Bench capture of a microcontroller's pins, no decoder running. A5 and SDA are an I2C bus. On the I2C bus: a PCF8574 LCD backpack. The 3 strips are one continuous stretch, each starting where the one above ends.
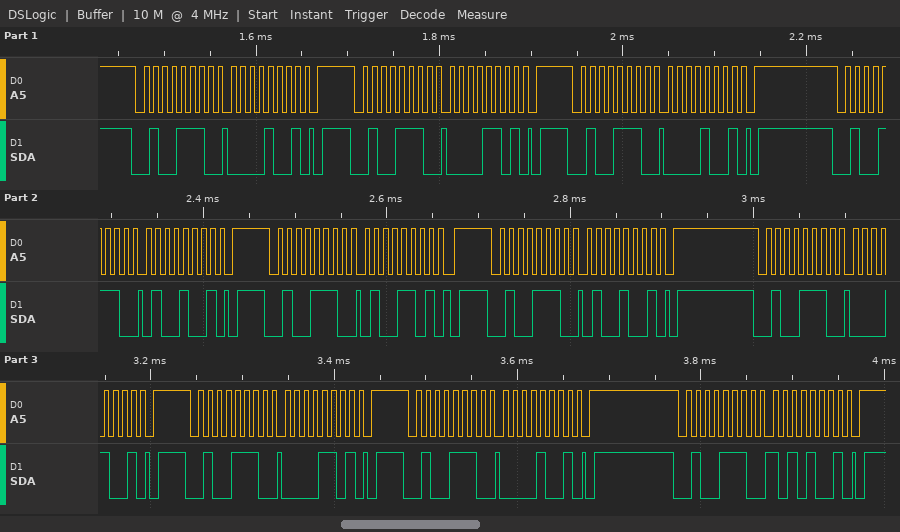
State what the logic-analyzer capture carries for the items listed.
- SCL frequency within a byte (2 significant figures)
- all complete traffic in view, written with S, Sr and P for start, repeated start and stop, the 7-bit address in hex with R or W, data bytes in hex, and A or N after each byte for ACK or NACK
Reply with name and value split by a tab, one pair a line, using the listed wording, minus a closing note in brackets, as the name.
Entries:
SCL frequency within a byte	100 kHz
all complete traffic in view, written with S, Sr and P for start, repeated start and stop, the 7-bit address in hex with R or W, data bytes in hex, and A or N after each byte for ACK or NACK	S 27W A 09 A P S 27W A 0D A P S 27W A 09 A P S 27W A 49 A P S 27W A 4D A P S 27W A 49 A P S 27W A 09 A P S 27W A 0D A P S 27W A 09 A P S 27W A A9 A P
